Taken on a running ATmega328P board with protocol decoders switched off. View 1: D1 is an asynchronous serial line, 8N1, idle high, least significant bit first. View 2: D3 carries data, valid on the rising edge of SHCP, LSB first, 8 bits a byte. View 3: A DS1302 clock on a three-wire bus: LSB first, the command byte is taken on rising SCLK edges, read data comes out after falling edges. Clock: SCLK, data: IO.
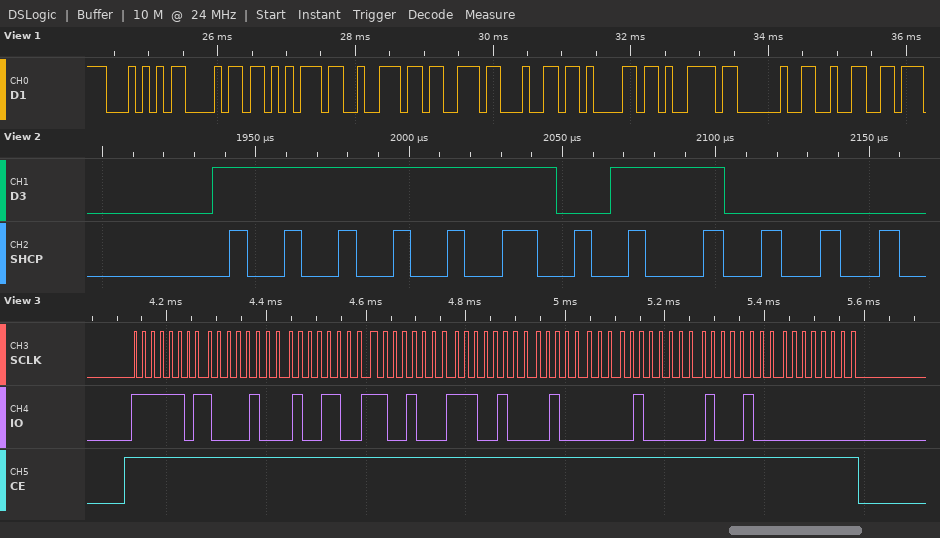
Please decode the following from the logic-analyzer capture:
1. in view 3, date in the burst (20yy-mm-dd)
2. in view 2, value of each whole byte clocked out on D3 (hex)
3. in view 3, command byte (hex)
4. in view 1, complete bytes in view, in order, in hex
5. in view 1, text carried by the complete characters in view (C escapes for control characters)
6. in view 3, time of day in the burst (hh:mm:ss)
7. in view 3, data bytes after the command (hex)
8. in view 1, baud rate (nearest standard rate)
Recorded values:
2022-04-27
BF
0xBF
54 68 75 72 73 64 61 79 20 32
"Thursday 2"
13:32:21
21 32 13 27 04 04 22 00
9600 baud
